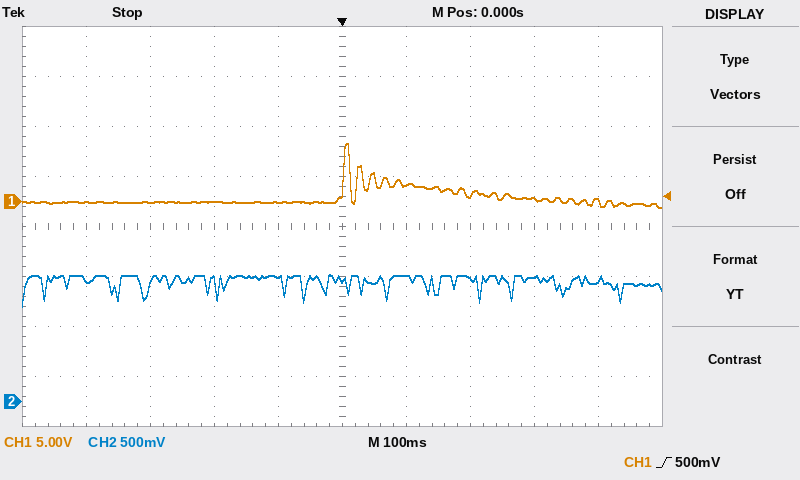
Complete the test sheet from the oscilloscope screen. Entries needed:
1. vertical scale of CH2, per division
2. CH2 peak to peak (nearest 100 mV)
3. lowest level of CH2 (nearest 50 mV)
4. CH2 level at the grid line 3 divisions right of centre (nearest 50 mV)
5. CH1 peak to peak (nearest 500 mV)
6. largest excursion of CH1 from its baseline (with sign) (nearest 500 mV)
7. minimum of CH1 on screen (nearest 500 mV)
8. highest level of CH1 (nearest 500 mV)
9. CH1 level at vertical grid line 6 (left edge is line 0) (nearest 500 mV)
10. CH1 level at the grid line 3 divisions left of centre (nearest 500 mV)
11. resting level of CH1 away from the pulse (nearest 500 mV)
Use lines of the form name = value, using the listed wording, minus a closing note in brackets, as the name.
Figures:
vertical scale of CH2, per division = 500 mV
CH2 peak to peak = 300 mV
lowest level of CH2 = 950 mV
CH2 level at the grid line 3 divisions right of centre = 1.25 V
CH1 peak to peak = 6.5 V
largest excursion of CH1 from its baseline (with sign) = +6.0 V
minimum of CH1 on screen = -500 mV
highest level of CH1 = 6.0 V
CH1 level at vertical grid line 6 (left edge is line 0) = 1.5 V
CH1 level at the grid line 3 divisions left of centre = 0.0 V
resting level of CH1 away from the pulse = 0.0 V
